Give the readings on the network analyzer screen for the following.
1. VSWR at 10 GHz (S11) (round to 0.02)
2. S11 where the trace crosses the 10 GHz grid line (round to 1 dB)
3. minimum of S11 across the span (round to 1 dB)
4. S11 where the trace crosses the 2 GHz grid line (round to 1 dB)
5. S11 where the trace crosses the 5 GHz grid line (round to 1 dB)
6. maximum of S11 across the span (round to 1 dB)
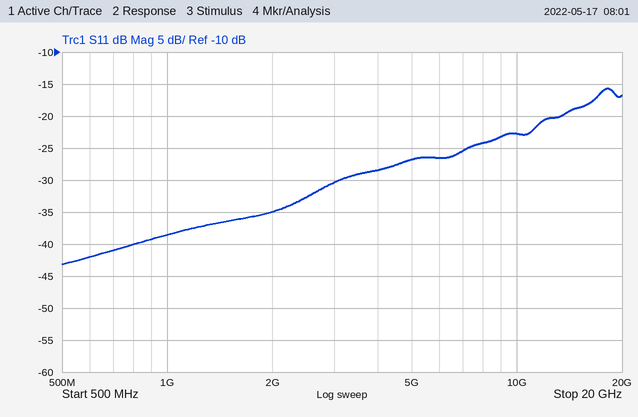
1.16
-23 dB
-43 dB
-35 dB
-27 dB
-16 dB
